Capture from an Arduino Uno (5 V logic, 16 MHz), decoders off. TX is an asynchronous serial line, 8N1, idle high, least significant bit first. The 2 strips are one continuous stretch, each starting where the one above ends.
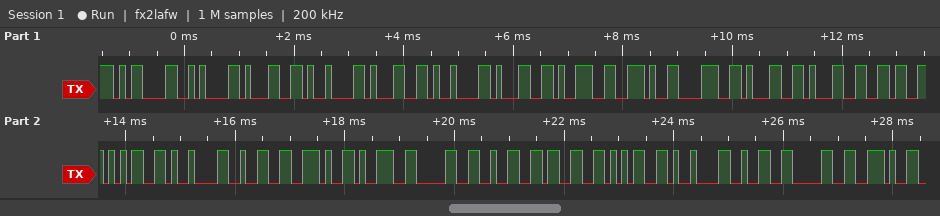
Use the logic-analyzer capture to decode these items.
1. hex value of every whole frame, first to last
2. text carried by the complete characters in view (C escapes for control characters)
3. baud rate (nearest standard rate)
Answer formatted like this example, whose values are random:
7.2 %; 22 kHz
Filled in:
0D 0A 31 09 31 09 31 39 2E 38 31 31 36 35 09 32 2E 39 30 32 33 35 09 32 30 2E; "\r\n1\t1\t19.81165\t2.90235\t20."; 9600 baud
